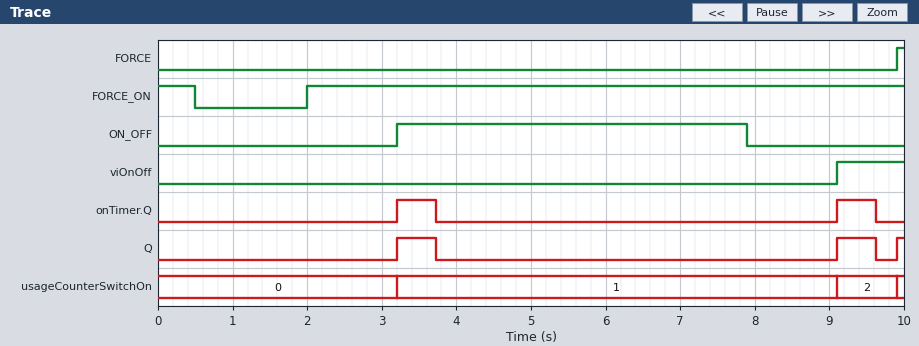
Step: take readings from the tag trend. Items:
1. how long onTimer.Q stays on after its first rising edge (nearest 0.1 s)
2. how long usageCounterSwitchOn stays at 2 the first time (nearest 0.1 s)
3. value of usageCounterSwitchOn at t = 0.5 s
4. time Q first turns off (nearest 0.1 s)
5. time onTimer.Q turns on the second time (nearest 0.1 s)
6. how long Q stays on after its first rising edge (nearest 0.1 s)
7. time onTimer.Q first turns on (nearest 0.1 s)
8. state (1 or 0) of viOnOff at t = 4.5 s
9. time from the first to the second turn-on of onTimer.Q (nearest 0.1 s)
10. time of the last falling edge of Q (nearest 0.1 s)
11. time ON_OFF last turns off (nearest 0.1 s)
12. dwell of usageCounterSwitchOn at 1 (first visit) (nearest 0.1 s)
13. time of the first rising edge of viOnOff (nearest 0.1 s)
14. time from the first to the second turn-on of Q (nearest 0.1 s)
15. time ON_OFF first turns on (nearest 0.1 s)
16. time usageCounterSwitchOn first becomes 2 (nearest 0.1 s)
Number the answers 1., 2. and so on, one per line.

1. 0.5 s
2. 0.8 s
3. 0
4. 3.7 s
5. 9.1 s
6. 0.5 s
7. 3.2 s
8. 0
9. 5.9 s
10. 9.6 s
11. 7.9 s
12. 5.9 s
13. 9.1 s
14. 5.9 s
15. 3.2 s
16. 9.1 s
